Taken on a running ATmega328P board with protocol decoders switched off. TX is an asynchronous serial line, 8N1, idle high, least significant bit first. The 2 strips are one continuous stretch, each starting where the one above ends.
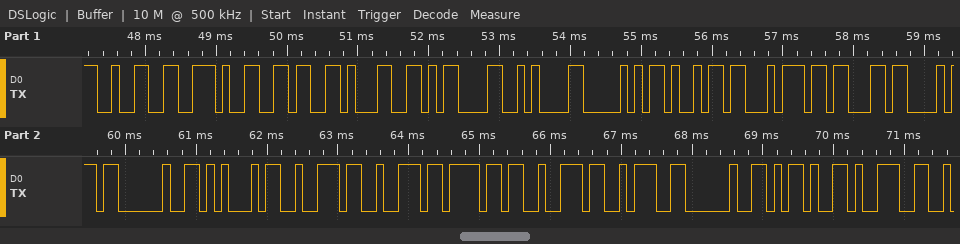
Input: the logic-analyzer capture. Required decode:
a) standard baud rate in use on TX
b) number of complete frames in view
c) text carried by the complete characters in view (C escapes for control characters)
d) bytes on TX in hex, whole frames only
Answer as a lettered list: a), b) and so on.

a) 9600 baud
b) 21
c) "2.61\r\nPitch Error: -9"
d) 32 2E 36 31 0D 0A 50 69 74 63 68 20 45 72 72 6F 72 3A 20 2D 39
